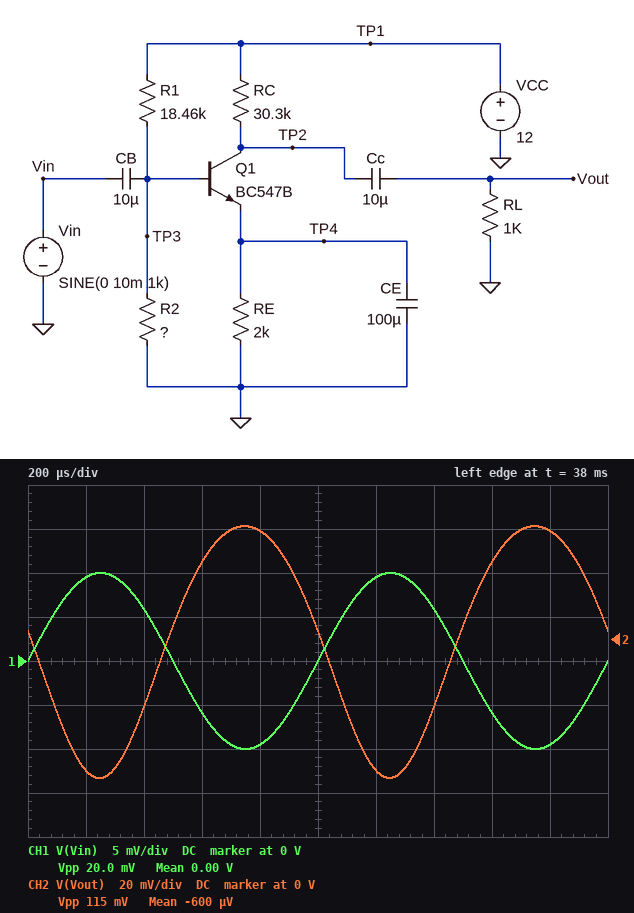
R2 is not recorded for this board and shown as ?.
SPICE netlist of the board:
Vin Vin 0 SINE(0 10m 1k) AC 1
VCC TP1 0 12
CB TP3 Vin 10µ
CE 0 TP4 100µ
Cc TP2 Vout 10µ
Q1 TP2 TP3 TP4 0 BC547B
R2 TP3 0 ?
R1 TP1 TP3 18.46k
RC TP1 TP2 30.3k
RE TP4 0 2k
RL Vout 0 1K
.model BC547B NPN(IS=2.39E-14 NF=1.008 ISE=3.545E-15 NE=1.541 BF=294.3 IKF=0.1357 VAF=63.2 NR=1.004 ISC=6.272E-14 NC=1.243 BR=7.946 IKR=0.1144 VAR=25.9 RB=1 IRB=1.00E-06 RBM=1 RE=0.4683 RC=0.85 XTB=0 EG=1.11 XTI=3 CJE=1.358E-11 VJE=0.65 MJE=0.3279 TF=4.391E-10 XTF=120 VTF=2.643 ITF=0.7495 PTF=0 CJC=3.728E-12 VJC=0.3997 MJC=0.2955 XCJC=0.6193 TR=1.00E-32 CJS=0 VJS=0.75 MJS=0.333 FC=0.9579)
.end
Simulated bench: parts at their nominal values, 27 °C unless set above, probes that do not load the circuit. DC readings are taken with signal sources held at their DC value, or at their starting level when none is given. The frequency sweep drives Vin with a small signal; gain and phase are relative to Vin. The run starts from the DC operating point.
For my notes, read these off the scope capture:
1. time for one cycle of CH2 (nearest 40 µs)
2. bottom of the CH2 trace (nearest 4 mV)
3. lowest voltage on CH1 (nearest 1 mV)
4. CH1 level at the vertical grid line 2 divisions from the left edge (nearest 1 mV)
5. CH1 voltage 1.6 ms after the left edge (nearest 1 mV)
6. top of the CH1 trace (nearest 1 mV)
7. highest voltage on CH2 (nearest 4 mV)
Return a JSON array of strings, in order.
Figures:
["1.00 ms", "-64 mV", "-10 mV", "6 mV", "-6 mV", "10 mV", "52 mV"]
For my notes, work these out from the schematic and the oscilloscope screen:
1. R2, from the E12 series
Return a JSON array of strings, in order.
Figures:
["1.5 kΩ"]
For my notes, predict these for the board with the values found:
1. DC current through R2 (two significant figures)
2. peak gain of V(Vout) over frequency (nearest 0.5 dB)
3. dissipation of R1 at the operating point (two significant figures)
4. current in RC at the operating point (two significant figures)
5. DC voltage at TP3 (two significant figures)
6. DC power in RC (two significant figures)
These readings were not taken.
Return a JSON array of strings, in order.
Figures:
["600 µA", "15.0 dB", "6.7 mW", "160 µA", "900 mV", "740 µW"]
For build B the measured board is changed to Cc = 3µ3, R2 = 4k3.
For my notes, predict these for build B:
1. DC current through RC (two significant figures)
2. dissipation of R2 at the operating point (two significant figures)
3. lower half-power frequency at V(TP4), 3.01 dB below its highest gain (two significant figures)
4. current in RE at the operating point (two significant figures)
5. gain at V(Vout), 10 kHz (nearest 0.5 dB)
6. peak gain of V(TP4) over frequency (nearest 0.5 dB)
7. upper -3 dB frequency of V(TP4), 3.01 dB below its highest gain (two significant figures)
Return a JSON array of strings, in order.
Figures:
["360 µA", "670 µW", "1.1 Hz", "520 µA", "-11.0 dB", "-21.5 dB", "160 Hz"]
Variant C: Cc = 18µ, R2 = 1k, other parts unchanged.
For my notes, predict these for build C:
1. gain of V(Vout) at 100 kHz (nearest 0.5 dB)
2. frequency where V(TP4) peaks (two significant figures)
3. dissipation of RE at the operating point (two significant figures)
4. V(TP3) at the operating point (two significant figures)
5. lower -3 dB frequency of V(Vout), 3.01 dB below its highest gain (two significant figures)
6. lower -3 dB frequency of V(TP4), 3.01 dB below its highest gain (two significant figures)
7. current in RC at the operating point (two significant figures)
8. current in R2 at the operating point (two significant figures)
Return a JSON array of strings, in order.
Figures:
["2.0 dB", "7.0 Hz", "2.4 µW", "620 mV", "17 Hz", "2.2 Hz", "35 µA", "620 µA"]
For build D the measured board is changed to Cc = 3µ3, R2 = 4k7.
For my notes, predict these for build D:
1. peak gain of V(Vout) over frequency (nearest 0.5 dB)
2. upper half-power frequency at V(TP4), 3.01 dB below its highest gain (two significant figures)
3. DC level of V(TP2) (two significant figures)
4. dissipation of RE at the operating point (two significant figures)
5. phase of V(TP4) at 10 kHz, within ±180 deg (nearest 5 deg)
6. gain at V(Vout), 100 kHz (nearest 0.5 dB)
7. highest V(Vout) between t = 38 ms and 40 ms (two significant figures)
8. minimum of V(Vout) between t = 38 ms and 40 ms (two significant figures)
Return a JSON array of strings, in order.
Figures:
["-0.5 dB", "170 Hz", "1.1 V", "590 µW", "-90 deg", "-12.0 dB", "3.0 mV", "-2.4 mV"]
